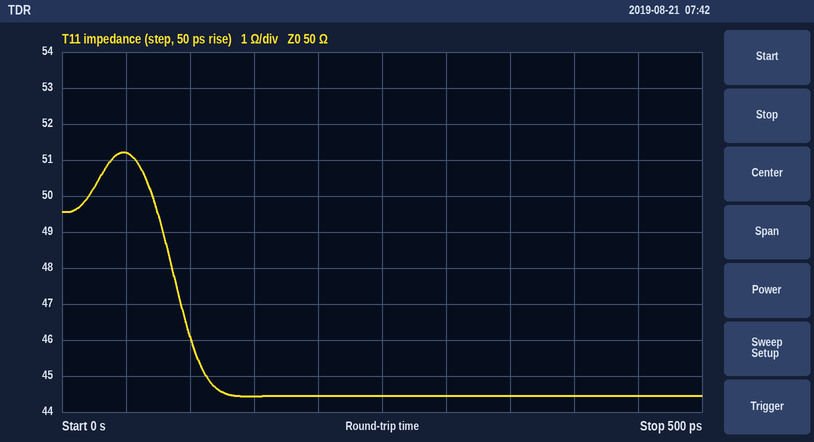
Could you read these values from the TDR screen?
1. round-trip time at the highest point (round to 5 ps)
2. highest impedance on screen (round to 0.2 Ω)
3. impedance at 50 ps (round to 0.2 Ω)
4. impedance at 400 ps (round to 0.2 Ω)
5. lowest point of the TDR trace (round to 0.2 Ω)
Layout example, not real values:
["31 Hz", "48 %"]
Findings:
["50 ps", "51.2 Ω", "51.2 Ω", "44.4 Ω", "44.4 Ω"]
